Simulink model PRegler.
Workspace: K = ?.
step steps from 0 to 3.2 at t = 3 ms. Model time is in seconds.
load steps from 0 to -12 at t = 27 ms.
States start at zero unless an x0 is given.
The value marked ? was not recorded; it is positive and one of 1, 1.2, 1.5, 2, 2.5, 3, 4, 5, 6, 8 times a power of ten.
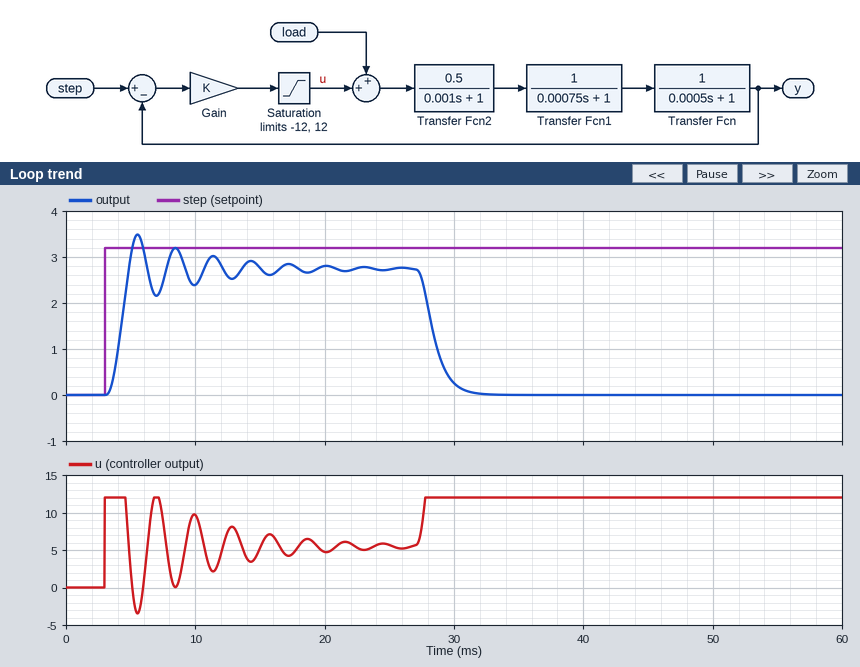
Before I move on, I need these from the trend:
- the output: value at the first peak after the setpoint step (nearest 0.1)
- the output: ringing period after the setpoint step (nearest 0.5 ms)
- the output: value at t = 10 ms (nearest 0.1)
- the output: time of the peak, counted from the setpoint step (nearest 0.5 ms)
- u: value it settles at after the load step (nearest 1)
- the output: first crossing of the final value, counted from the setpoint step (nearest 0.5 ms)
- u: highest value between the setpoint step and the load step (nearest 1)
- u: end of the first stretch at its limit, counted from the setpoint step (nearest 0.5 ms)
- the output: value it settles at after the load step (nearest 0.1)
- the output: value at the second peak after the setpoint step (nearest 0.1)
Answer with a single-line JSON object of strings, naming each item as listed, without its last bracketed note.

{"the output: value at the first peak after the setpoint step": "3.5", "the output: ringing period after the setpoint step": "3.0 ms", "the output: value at t = 10 ms": "2.4", "the output: time of the peak, counted from the setpoint step": "2.5 ms", "u: value it settles at after the load step": "12", "the output: first crossing of the final value, counted from the setpoint step": "2.0 ms", "u: highest value between the setpoint step and the load step": "12", "u: end of the first stretch at its limit, counted from the setpoint step": "1.5 ms", "the output: value it settles at after the load step": "0.0", "the output: value at the second peak after the setpoint step": "3.2"}
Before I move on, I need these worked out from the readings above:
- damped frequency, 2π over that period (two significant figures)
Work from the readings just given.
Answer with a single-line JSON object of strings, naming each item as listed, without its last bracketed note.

{"damped frequency, 2π over that period": "2.1 rad/ms"}
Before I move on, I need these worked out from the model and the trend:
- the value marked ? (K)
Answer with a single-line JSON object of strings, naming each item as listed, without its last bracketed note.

{"the value marked ?": "12"}
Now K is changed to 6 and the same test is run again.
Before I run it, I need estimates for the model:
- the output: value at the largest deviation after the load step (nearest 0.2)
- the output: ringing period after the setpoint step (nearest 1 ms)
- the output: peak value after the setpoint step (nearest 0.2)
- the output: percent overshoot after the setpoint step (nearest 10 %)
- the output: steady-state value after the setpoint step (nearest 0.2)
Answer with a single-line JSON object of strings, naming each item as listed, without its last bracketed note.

{"the output: value at the largest deviation after the load step": "-0.2", "the output: ringing period after the setpoint step": "4 ms", "the output: peak value after the setpoint step": "3.2", "the output: percent overshoot after the setpoint step": "30 %", "the output: steady-state value after the setpoint step": "2.4"}
